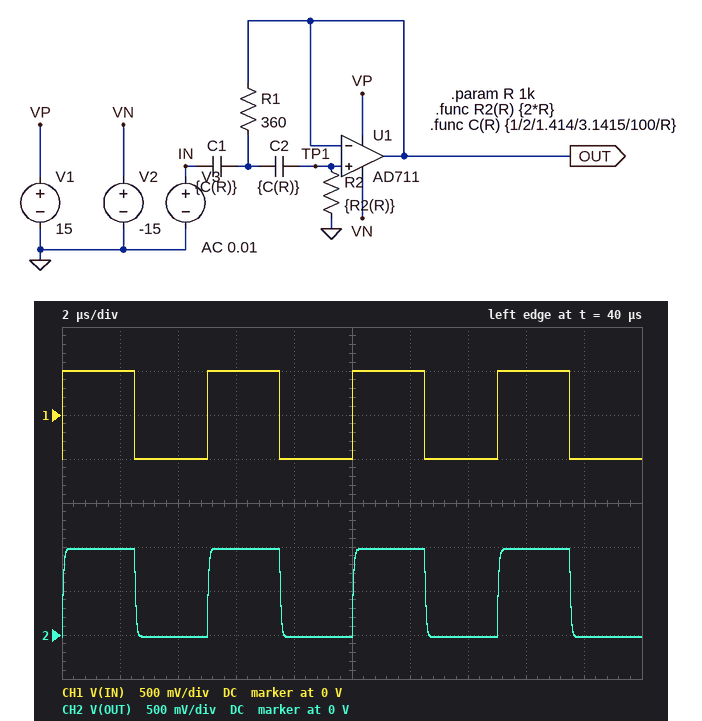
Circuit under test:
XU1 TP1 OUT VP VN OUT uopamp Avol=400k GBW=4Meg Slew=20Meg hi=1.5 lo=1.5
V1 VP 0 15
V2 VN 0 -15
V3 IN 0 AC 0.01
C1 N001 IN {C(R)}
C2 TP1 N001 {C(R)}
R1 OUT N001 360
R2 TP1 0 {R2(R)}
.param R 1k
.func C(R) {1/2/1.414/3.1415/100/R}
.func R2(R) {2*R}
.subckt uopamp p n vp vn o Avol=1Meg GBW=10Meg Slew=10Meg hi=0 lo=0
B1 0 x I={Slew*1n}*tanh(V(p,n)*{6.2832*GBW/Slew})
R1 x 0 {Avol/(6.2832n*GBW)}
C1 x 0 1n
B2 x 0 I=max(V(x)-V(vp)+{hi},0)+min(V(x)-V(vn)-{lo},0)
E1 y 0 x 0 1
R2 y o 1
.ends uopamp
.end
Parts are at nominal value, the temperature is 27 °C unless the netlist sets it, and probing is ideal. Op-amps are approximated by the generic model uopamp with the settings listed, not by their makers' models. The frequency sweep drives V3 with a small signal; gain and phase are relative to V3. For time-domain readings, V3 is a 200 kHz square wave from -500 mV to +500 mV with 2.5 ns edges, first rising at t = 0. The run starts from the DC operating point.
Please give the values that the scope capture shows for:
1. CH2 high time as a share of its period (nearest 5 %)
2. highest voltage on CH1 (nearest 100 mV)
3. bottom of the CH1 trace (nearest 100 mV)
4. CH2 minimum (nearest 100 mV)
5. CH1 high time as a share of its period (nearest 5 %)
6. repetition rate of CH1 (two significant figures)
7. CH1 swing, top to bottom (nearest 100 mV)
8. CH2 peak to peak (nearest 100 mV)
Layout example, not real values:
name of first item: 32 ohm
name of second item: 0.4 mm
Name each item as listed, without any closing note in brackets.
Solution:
CH2 high time as a share of its period: 50 %
highest voltage on CH1: 500 mV
bottom of the CH1 trace: -500 mV
CH2 minimum: 0 V
CH1 high time as a share of its period: 50 %
repetition rate of CH1: 200 kHz
CH1 swing, top to bottom: 1.0 V
CH2 peak to peak: 1.0 V
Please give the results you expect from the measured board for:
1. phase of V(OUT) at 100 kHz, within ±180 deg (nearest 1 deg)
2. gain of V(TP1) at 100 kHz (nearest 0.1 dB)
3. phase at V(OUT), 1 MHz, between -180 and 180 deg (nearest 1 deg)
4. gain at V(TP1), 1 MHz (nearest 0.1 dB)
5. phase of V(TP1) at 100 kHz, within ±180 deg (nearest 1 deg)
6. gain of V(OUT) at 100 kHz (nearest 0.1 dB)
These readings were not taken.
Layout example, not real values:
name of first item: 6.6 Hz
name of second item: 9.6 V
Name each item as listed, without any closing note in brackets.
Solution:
phase of V(OUT) at 100 kHz, within ±180 deg: -1 deg
gain of V(TP1) at 100 kHz: 0 dB
phase at V(OUT), 1 MHz, between -180 and 180 deg: -14 deg
gain at V(TP1), 1 MHz: 0 dB
phase of V(TP1) at 100 kHz, within ±180 deg: 0 deg
gain of V(OUT) at 100 kHz: 0 dB
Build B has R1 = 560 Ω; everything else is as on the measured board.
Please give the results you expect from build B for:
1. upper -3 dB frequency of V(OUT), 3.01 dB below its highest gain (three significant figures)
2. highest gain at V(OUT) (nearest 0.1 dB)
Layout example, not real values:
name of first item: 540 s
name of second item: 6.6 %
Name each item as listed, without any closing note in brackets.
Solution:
upper -3 dB frequency of V(OUT), 3.01 dB below its highest gain: 3.13 MHz
highest gain at V(OUT): 0.9 dB
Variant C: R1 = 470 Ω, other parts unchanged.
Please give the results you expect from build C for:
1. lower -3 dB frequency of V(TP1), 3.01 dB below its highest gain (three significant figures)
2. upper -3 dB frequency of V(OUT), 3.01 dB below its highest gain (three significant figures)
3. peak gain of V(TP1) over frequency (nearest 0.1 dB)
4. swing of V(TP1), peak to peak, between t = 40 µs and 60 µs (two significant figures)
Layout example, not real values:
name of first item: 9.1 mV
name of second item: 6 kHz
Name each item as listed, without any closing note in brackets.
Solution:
lower -3 dB frequency of V(TP1), 3.01 dB below its highest gain: 124 Hz
upper -3 dB frequency of V(OUT), 3.01 dB below its highest gain: 2.64 MHz
peak gain of V(TP1) over frequency: 1.4 dB
swing of V(TP1), peak to peak, between t = 40 µs and 60 µs: 1.0 V
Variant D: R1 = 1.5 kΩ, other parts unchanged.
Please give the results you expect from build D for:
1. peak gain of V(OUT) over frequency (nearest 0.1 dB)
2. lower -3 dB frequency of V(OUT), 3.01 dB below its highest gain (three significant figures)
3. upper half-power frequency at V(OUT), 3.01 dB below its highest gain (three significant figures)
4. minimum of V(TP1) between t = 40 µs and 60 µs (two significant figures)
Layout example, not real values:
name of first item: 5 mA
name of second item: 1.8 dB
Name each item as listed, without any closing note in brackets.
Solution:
peak gain of V(OUT) over frequency: 0 dB
lower -3 dB frequency of V(OUT), 3.01 dB below its highest gain: 104 Hz
upper half-power frequency at V(OUT), 3.01 dB below its highest gain: 4.00 MHz
minimum of V(TP1) between t = 40 µs and 60 µs: -26 mV
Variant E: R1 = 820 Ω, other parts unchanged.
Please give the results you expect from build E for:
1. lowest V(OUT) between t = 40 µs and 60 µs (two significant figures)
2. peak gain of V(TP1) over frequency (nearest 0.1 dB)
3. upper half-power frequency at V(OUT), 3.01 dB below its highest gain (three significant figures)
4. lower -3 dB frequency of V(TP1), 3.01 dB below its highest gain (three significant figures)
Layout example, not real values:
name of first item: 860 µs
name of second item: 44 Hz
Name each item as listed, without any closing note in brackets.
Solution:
lowest V(OUT) between t = 40 µs and 60 µs: -26 mV
peak gain of V(TP1) over frequency: 0.1 dB
upper half-power frequency at V(OUT), 3.01 dB below its highest gain: 3.86 MHz
lower -3 dB frequency of V(TP1), 3.01 dB below its highest gain: 102 Hz
